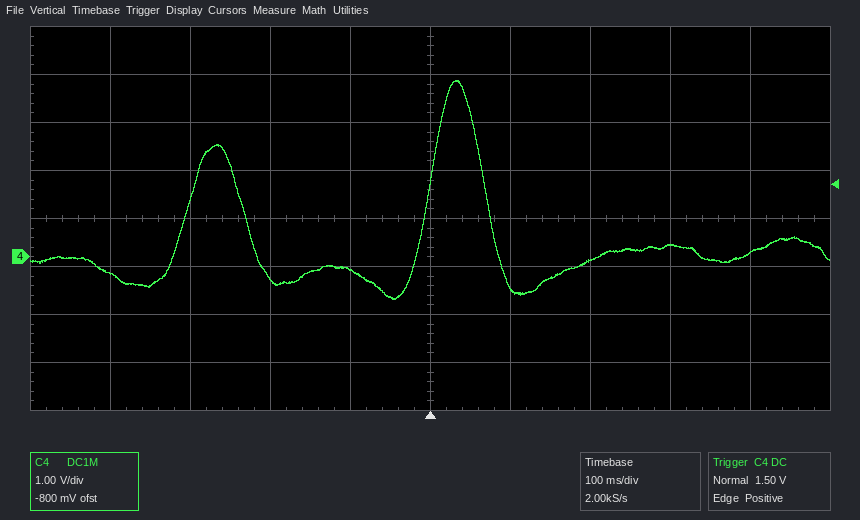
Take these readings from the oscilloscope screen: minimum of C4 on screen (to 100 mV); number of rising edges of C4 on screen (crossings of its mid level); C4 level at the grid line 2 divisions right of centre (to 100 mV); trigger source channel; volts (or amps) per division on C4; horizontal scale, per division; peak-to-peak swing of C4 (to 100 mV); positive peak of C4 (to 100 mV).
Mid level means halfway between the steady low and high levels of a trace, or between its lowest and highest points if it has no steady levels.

-900 mV
2
-100 mV
C4
1 V
100 ms
4.6 V
3.7 V
